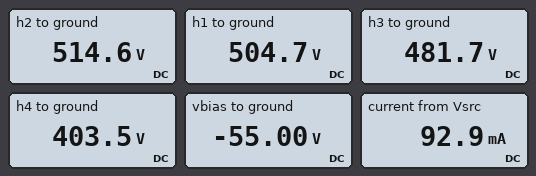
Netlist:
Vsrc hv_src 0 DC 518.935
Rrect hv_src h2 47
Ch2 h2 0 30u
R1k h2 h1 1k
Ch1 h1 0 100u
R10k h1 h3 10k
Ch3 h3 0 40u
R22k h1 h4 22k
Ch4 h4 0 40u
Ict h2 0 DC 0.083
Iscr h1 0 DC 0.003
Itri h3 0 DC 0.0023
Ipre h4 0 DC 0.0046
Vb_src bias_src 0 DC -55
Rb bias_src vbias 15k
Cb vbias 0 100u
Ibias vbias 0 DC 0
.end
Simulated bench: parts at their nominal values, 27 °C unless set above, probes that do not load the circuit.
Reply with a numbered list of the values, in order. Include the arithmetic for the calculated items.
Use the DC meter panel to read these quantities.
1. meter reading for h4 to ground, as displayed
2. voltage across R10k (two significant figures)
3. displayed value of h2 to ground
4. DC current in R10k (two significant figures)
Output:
1. 403.5 V
2. 504.7 V - 481.7 V = 23 V
3. 514.6 V
4. (504.7 V - 481.7 V) / 10 kΩ = 2.3 mA
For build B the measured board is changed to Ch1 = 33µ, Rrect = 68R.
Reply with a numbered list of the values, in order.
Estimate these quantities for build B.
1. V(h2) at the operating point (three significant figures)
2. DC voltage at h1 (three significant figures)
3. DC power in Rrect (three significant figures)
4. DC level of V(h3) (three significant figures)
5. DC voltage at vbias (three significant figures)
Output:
1. 513 V
2. 503 V
3. 587 mW
4. 480 V
5. -55.0 V
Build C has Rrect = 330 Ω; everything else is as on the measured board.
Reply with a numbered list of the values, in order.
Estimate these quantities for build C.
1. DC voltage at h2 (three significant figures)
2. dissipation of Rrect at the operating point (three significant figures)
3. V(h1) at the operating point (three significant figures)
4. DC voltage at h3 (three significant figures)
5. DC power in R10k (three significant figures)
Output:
1. 488 V
2. 2.85 W
3. 478 V
4. 455 V
5. 52.9 mW
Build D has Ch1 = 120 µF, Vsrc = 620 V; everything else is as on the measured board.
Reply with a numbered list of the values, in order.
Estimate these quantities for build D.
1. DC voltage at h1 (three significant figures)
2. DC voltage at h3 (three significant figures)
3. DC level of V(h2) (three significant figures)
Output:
1. 606 V
2. 583 V
3. 616 V
